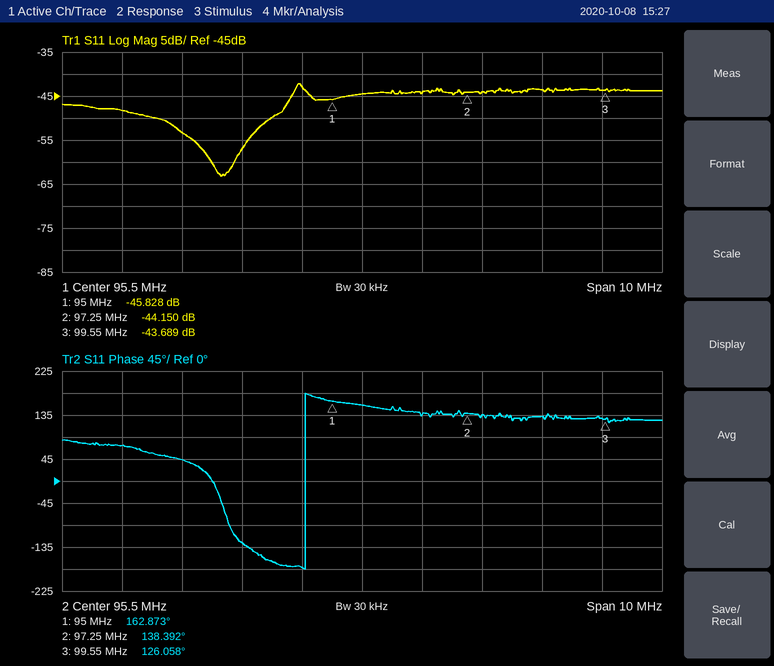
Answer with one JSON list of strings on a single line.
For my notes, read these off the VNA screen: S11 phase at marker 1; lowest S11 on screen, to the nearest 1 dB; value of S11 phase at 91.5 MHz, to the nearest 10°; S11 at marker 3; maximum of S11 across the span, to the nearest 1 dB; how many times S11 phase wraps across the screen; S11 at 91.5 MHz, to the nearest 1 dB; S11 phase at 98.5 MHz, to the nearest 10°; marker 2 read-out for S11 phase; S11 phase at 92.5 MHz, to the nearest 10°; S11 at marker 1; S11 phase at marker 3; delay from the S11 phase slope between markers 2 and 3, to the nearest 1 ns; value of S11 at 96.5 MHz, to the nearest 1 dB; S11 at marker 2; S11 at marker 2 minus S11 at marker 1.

["162.873°", "-63 dB", "70°", "-43.689 dB", "-42 dB", "1", "-48 dB", "130°", "138.392°", "40°", "-45.828 dB", "126.058°", "15 ns", "-44 dB", "-44.150 dB", "1.678 dB"]
